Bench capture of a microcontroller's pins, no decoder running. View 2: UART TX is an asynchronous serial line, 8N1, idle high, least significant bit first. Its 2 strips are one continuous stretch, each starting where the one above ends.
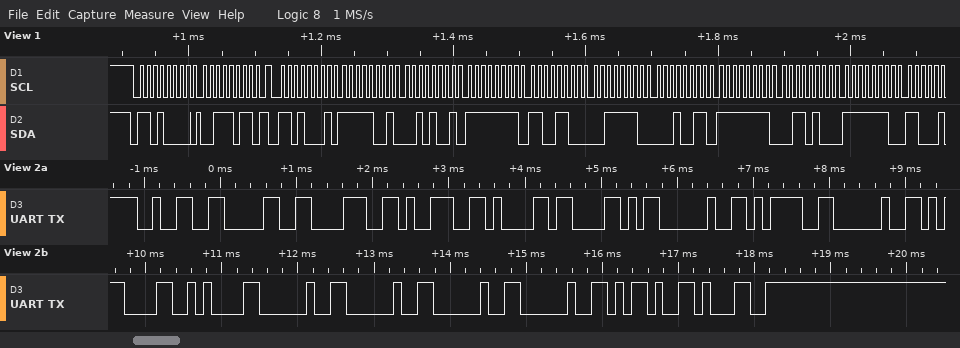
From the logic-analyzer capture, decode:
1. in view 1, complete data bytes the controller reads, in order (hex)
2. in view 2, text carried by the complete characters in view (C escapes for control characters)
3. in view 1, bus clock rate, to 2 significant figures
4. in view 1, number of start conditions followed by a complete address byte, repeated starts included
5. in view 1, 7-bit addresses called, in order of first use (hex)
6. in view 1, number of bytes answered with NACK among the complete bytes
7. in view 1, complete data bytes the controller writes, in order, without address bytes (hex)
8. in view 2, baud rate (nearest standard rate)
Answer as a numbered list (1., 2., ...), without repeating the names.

1. F9 29 FF CC 3E 13 FF 34 FE
2. "2089aX = \r\n    -1"
3. 100 kHz
4. 2
5. 0x68
6. 0
7. 3B
8. 9600 baud
